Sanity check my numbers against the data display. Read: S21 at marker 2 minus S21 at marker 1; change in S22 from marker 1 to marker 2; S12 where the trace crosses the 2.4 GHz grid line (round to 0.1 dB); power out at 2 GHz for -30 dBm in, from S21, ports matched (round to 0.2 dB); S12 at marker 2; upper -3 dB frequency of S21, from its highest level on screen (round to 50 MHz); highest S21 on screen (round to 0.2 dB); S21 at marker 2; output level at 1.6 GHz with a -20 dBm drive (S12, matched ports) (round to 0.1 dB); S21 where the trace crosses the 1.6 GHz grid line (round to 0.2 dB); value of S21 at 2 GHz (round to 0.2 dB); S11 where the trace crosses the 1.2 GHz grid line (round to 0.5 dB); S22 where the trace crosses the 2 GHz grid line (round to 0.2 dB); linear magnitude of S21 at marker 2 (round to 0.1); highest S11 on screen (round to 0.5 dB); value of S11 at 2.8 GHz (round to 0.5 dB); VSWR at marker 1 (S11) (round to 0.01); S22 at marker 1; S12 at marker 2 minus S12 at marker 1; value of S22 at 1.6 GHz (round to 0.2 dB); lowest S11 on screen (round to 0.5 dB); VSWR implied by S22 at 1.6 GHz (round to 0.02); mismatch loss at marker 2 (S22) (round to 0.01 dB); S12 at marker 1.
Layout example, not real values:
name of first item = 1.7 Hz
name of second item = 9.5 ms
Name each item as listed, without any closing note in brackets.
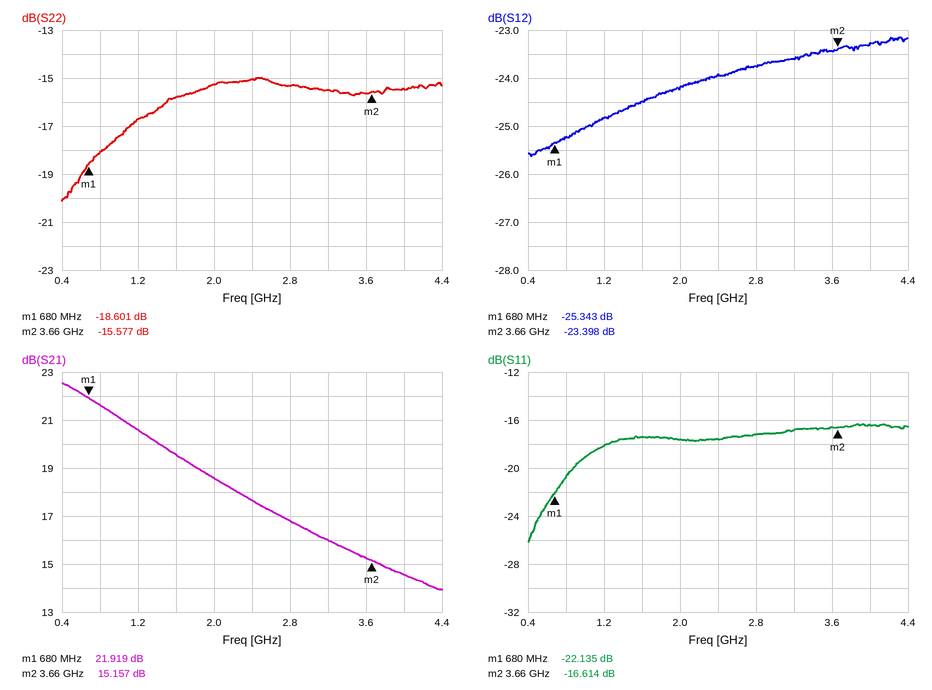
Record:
S21 at marker 2 minus S21 at marker 1 = -6.762 dB
change in S22 from marker 1 to marker 2 = 3.024 dB
S12 where the trace crosses the 2.4 GHz grid line = -23.9 dB
power out at 2 GHz for -30 dBm in, from S21, ports matched = -11.4 dBm
S12 at marker 2 = -23.398 dB
upper -3 dB frequency of S21, from its highest level on screen = 1.60 GHz
highest S21 on screen = 22.6 dB
S21 at marker 2 = 15.157 dB
output level at 1.6 GHz with a -20 dBm drive (S12, matched ports) = -44.5 dBm
S21 where the trace crosses the 1.6 GHz grid line = 19.6 dB
value of S21 at 2 GHz = 18.6 dB
S11 where the trace crosses the 1.2 GHz grid line = -18.0 dB
S22 where the trace crosses the 2 GHz grid line = -15.2 dB
linear magnitude of S21 at marker 2 = 5.7
highest S11 on screen = -16.5 dB
value of S11 at 2.8 GHz = -17.0 dB
VSWR at marker 1 (S11) = 1.17
S22 at marker 1 = -18.601 dB
S12 at marker 2 minus S12 at marker 1 = 1.945 dB
value of S22 at 1.6 GHz = -15.8 dB
lowest S11 on screen = -26.0 dB
VSWR implied by S22 at 1.6 GHz = 1.38
mismatch loss at marker 2 (S22) = 0.12 dB
S12 at marker 1 = -25.343 dB
